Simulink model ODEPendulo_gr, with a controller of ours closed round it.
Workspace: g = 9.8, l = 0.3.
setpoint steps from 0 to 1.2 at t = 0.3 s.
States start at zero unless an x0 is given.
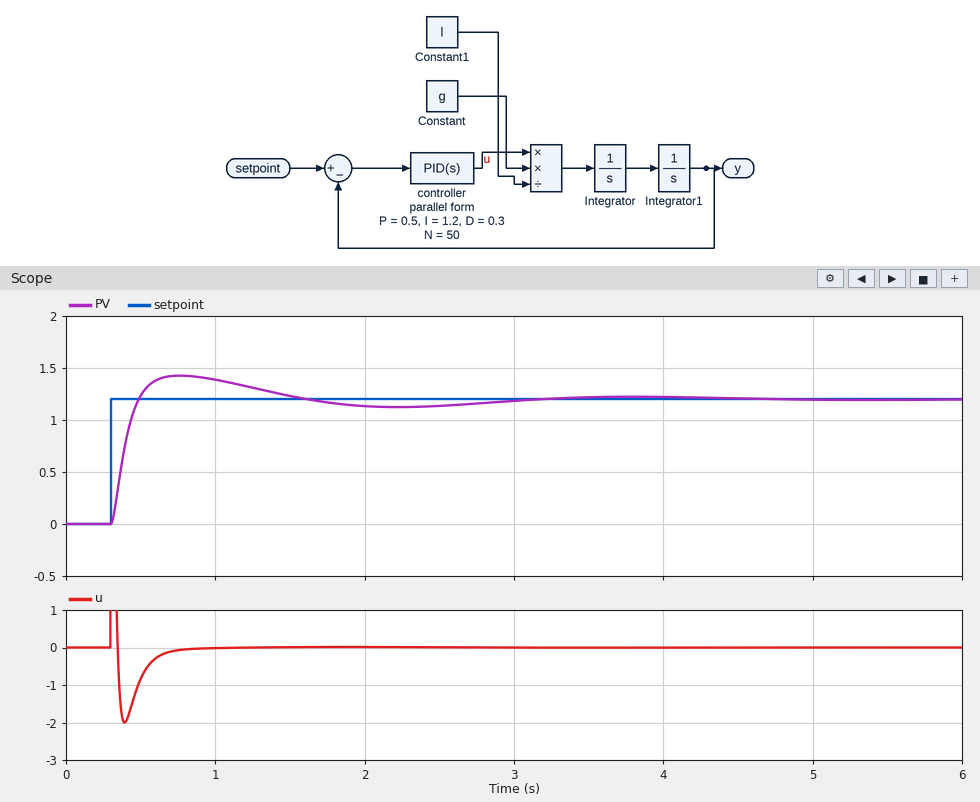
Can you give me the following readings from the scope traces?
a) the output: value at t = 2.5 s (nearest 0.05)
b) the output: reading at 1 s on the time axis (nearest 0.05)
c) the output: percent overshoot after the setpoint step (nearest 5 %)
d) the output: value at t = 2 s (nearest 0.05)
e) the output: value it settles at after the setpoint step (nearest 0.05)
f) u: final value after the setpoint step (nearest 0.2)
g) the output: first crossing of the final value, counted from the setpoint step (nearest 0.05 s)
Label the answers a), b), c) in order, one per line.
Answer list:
a) 1.15
b) 1.40
c) 20 %
d) 1.15
e) 1.20
f) 0.0
g) 0.20 s
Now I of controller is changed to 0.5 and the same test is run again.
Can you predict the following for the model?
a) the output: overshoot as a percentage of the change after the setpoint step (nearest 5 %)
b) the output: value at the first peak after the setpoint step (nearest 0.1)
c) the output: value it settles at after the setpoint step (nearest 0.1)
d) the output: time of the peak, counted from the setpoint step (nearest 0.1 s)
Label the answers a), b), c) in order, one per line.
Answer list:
a) 15 %
b) 1.4
c) 1.2
d) 0.4 s
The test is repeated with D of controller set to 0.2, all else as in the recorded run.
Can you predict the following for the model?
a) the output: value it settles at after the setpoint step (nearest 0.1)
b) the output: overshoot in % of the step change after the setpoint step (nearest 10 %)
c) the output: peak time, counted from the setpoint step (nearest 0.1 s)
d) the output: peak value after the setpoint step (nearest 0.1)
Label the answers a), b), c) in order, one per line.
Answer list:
a) 1.2
b) 30 %
c) 0.5 s
d) 1.6
